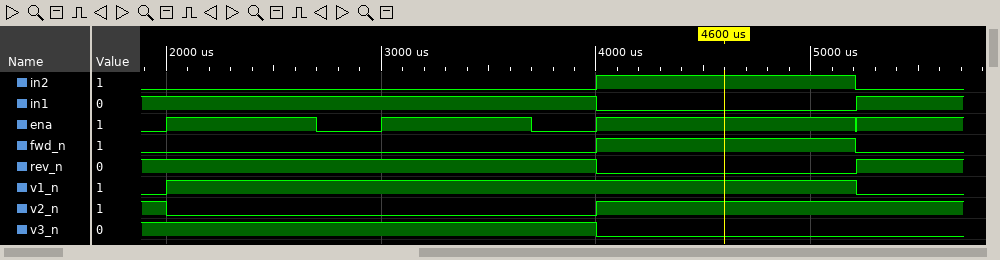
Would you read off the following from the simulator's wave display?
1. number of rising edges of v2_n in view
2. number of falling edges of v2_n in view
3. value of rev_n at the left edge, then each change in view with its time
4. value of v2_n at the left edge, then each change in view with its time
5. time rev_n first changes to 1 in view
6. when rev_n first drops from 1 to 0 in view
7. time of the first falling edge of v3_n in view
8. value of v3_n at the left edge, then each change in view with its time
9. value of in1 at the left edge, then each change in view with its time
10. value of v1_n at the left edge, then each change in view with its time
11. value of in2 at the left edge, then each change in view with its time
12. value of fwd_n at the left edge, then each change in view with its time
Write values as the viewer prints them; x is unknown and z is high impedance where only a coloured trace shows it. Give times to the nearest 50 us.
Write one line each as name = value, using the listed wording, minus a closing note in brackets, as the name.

number of rising edges of v2_n in view = 1
number of falling edges of v2_n in view = 1
value of rev_n at the left edge, then each change in view with its time = 1, 0 at 4000 us, 1 at 5200 us
value of v2_n at the left edge, then each change in view with its time = 1, 0 at 2000 us, 1 at 4000 us
time rev_n first changes to 1 in view = 5200 us
when rev_n first drops from 1 to 0 in view = 4000 us
time of the first falling edge of v3_n in view = 4000 us
value of v3_n at the left edge, then each change in view with its time = 1, 0 at 4000 us
value of in1 at the left edge, then each change in view with its time = 1, 0 at 4000 us, 1 at 5200 us
value of v1_n at the left edge, then each change in view with its time = 0, 1 at 2000 us, 0 at 5200 us
value of in2 at the left edge, then each change in view with its time = 0, 1 at 4000 us, 0 at 5200 us
value of fwd_n at the left edge, then each change in view with its time = 0, 1 at 4000 us, 0 at 5200 us
